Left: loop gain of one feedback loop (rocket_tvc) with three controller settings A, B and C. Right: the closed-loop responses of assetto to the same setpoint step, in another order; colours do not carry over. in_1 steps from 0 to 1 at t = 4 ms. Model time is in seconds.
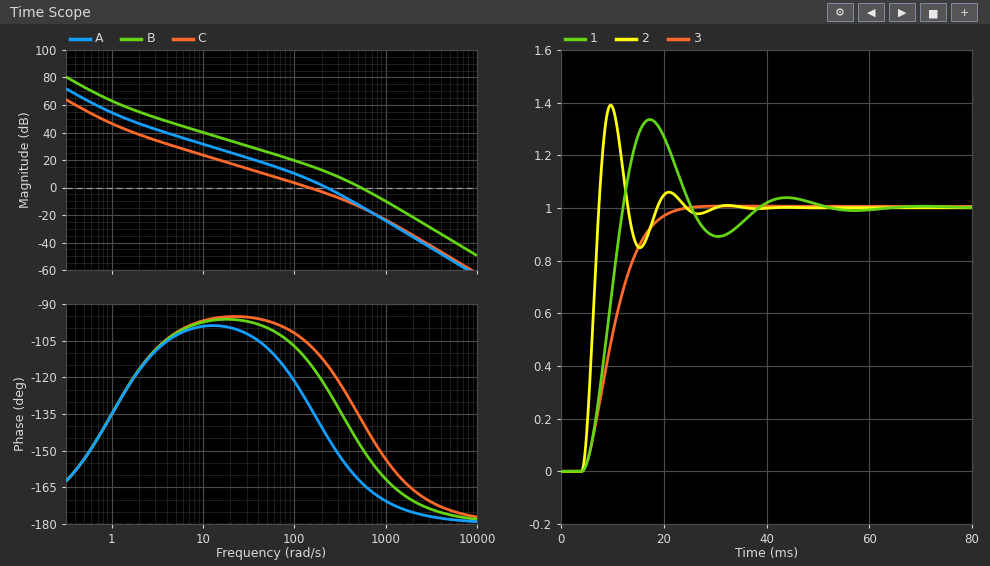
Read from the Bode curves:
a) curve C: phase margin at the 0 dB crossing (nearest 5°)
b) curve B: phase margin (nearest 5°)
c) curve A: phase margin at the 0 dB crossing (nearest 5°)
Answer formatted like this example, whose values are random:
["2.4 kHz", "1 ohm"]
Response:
["75°", "30°", "35°"]
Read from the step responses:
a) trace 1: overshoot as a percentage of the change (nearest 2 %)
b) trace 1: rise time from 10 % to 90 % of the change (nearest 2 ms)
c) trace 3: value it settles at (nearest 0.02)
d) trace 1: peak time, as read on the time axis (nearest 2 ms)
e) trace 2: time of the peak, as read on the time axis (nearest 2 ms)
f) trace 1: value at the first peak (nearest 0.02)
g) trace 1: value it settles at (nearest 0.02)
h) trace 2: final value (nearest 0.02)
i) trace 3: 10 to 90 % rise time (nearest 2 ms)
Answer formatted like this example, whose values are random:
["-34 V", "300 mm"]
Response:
["34 %", "6 ms", "1.00", "18 ms", "10 ms", "1.34", "1.00", "1.00", "10 ms"]
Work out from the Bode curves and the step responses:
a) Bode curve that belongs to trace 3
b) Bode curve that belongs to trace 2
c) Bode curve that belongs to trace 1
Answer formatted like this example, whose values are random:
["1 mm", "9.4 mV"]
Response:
["C", "B", "A"]
